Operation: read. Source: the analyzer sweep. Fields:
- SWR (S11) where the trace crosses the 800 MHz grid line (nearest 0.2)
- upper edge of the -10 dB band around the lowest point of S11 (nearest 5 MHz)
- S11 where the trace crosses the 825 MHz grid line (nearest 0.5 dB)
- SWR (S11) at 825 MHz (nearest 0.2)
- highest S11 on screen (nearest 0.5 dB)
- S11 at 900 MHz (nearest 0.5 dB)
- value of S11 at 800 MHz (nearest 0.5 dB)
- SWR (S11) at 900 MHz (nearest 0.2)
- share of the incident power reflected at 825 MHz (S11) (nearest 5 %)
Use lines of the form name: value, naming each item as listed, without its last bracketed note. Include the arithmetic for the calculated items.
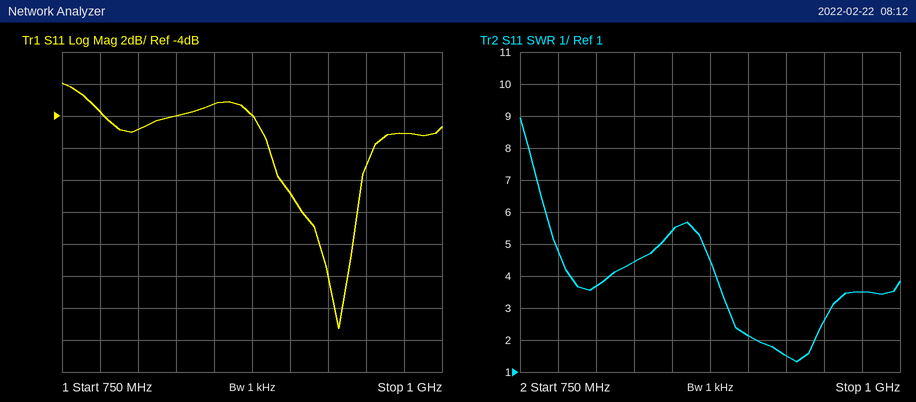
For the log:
SWR (S11) where the trace crosses the 800 MHz grid line: 3.6
upper edge of the -10 dB band around the lowest point of S11: 945 MHz
S11 where the trace crosses the 825 MHz grid line: -4.0 dB
SWR (S11) at 825 MHz: 4.4
highest S11 on screen: -2.0 dB
S11 at 900 MHz: -9.0 dB
value of S11 at 800 MHz: -5.0 dB
SWR (S11) at 900 MHz: 2.2
share of the incident power reflected at 825 MHz (S11): 10^(-4/10) ≈ 40 %
